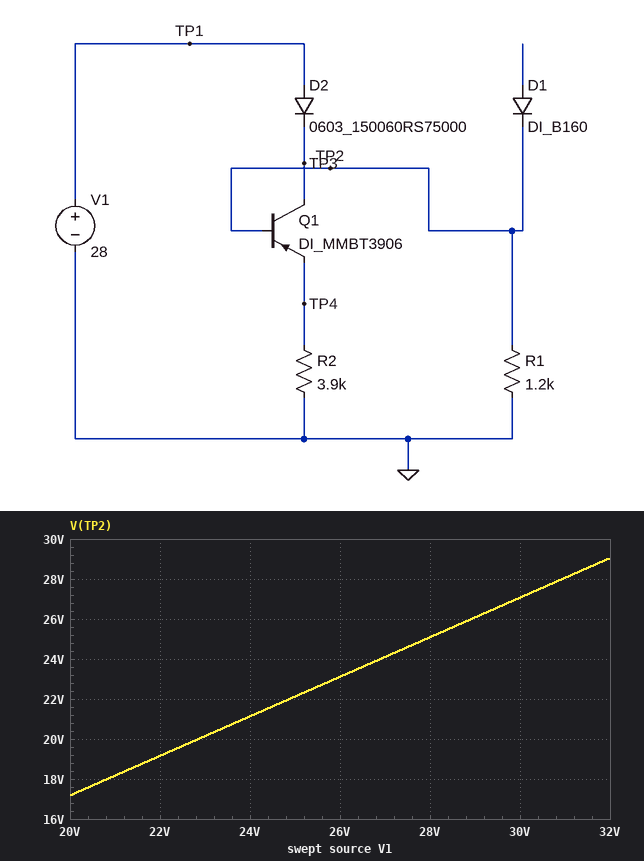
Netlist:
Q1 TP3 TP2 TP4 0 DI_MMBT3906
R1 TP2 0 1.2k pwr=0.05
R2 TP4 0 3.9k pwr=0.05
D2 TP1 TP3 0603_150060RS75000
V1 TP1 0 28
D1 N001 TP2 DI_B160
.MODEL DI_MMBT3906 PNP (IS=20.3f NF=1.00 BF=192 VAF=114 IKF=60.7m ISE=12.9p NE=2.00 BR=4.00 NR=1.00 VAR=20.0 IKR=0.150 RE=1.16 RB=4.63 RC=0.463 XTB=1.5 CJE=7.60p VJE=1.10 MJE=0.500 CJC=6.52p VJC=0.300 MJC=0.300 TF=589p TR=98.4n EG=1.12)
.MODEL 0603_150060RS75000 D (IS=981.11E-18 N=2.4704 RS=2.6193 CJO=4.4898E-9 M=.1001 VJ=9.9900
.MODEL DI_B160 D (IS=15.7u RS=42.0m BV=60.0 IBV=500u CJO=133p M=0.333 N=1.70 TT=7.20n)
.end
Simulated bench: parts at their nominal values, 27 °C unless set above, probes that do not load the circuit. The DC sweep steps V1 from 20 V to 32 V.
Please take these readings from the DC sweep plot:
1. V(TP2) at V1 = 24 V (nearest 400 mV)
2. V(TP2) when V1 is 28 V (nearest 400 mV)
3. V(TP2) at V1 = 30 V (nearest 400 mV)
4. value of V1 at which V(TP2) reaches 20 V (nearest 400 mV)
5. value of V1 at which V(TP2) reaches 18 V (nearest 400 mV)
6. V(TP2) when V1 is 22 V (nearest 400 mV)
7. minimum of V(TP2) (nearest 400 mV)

21.2 V
25.2 V
27.2 V
22.8 V
20.8 V
19.2 V
17.2 V
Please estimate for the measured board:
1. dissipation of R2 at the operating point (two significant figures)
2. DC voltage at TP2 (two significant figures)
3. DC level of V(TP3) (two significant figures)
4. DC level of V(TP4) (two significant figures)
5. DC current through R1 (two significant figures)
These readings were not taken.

170 mW
25 V
26 V
26 V
21 mA
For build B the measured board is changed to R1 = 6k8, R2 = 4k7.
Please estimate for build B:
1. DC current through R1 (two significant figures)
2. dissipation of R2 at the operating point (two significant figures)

3.7 mA
140 mW
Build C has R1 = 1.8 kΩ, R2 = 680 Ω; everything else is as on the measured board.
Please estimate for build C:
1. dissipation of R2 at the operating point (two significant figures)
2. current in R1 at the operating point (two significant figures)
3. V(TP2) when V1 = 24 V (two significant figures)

970 mW
14 mA
21 V
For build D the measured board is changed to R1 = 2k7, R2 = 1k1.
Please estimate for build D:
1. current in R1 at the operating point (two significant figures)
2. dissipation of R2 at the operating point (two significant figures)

9.3 mA
610 mW
